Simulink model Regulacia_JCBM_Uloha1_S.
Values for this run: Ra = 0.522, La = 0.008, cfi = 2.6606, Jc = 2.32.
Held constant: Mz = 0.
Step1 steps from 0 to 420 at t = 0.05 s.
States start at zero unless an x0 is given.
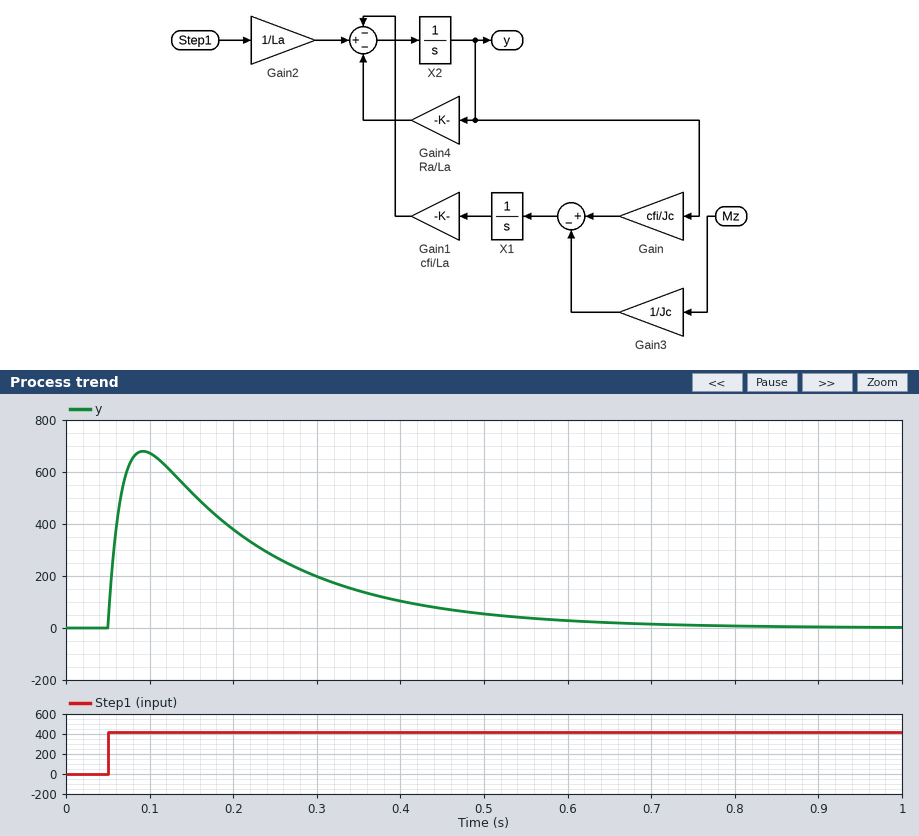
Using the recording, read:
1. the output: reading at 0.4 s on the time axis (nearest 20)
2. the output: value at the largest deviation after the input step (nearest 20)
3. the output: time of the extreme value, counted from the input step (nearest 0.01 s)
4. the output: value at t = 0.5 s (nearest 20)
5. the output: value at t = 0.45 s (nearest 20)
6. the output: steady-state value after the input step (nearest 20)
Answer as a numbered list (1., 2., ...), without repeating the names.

1. 100
2. 680
3. 0.04 s
4. 60
5. 80
6. 0
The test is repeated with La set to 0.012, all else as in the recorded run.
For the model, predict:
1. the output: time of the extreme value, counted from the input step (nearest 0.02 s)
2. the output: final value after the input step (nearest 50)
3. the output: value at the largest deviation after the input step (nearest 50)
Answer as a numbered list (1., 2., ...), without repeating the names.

1. 0.06 s
2. 0
3. 650
